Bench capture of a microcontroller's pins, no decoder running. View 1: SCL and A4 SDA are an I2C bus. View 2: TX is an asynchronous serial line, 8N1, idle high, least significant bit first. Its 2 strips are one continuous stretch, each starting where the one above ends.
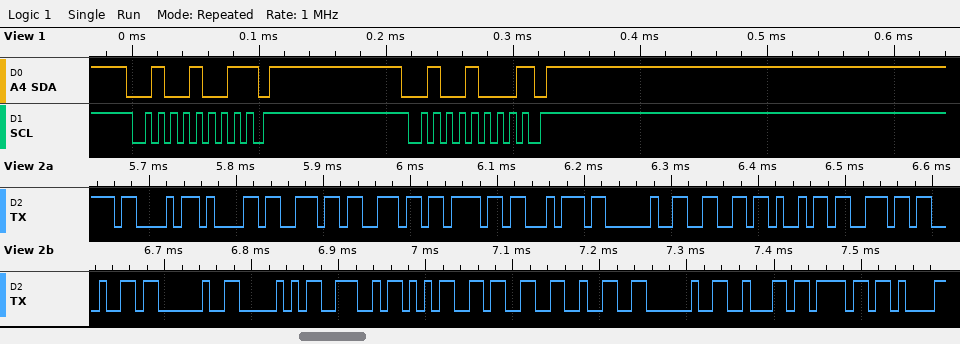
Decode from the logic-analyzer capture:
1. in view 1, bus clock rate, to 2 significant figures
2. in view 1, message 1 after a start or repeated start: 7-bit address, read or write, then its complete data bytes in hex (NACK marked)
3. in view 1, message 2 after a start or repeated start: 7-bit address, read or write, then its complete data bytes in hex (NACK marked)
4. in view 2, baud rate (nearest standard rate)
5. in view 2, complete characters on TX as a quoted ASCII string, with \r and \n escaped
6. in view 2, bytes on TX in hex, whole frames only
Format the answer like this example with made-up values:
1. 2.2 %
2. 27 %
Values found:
1. 100 kHz
2. 0x24 read NACK
3. 0x24 write NACK
4. 115200 baud
5. "Cannot find PN532 bo"
6. 0x43 0x61 0x6E 0x6E 0x6F 0x74 0x20 0x66 0x69 0x6E 0x64 0x20 0x50 0x4E 0x35 0x33 0x32 0x20 0x62 0x6F
